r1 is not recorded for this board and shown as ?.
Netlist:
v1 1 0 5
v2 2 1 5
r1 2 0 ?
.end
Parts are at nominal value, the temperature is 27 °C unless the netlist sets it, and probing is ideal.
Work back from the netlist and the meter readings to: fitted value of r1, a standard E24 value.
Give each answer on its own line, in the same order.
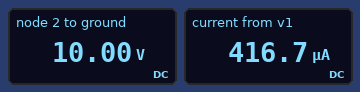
24 kΩ
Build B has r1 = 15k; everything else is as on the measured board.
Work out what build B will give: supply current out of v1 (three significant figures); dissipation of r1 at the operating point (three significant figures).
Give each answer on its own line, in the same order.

667 µA
6.67 mW
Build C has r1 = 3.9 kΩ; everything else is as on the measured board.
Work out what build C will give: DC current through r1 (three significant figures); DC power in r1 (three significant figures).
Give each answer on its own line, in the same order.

2.56 mA
25.6 mW
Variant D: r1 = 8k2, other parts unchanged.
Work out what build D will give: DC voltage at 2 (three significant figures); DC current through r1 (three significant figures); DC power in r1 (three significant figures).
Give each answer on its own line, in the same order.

10.0 V
1.22 mA
12.2 mW
